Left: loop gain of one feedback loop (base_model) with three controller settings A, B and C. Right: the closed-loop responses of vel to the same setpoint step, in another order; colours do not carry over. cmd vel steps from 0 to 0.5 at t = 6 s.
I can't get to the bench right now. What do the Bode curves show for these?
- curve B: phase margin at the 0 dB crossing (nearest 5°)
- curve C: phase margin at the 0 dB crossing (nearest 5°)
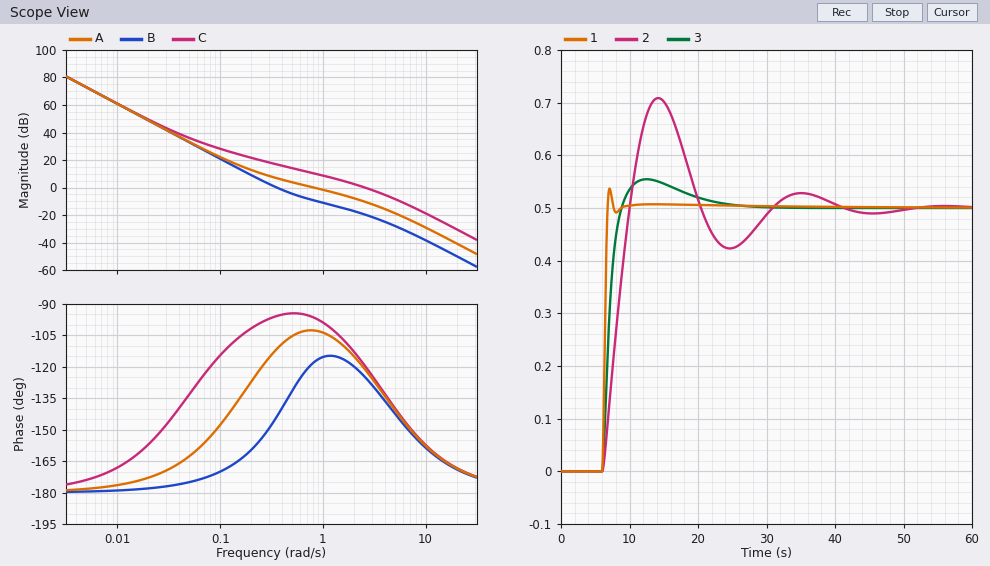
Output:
35°
60°
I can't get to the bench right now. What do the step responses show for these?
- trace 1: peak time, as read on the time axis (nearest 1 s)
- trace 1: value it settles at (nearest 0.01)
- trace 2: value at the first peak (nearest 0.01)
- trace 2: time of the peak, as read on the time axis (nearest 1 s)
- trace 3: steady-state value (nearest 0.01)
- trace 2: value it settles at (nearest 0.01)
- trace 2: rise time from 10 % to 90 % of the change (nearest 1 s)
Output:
7 s
0.50
0.71
14 s
0.50
0.50
3 s
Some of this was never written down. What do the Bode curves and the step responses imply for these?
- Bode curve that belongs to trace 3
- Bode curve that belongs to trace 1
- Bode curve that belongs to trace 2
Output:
A
C
B
